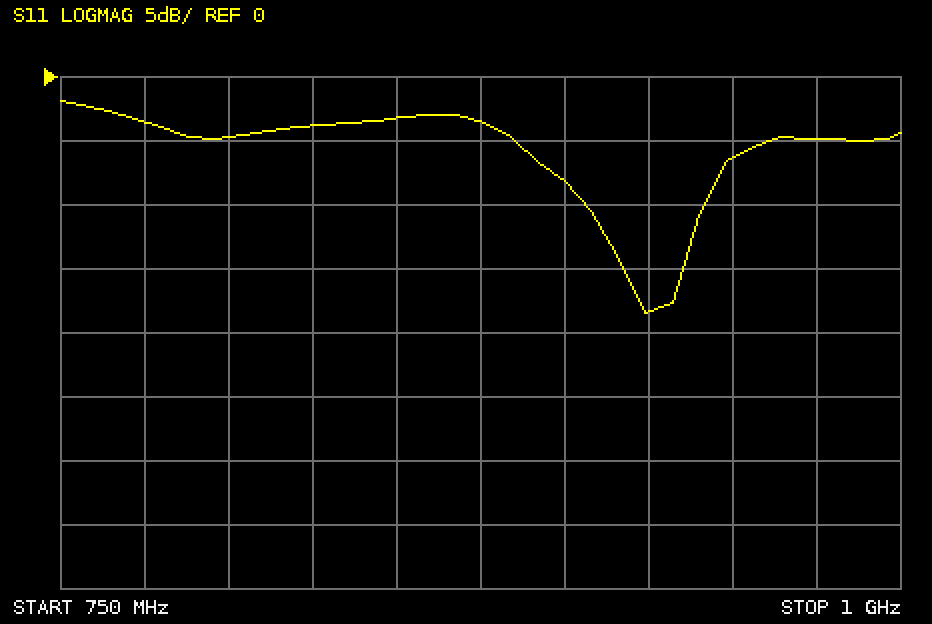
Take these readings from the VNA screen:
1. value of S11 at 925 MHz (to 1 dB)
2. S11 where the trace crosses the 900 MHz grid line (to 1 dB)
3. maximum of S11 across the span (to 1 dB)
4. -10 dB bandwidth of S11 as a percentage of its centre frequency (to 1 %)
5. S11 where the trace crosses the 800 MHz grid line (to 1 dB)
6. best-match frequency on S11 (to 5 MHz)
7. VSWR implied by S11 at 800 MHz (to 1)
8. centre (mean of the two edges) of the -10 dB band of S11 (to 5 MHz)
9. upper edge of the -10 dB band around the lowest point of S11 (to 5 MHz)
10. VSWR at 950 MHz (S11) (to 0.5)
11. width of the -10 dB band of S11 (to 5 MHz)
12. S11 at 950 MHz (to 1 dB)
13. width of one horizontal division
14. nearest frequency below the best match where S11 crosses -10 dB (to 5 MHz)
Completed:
-18 dB
-8 dB
-2 dB
4 %
-5 dB
925 MHz
4
925 MHz
940 MHz
3.0
35 MHz
-6 dB
25 MHz
905 MHz
